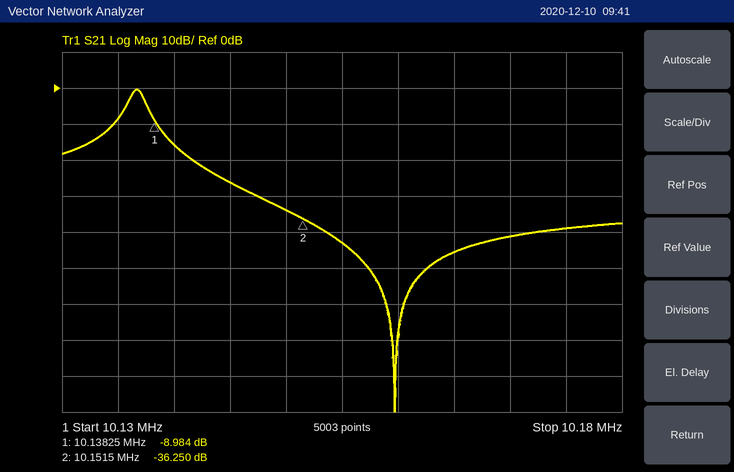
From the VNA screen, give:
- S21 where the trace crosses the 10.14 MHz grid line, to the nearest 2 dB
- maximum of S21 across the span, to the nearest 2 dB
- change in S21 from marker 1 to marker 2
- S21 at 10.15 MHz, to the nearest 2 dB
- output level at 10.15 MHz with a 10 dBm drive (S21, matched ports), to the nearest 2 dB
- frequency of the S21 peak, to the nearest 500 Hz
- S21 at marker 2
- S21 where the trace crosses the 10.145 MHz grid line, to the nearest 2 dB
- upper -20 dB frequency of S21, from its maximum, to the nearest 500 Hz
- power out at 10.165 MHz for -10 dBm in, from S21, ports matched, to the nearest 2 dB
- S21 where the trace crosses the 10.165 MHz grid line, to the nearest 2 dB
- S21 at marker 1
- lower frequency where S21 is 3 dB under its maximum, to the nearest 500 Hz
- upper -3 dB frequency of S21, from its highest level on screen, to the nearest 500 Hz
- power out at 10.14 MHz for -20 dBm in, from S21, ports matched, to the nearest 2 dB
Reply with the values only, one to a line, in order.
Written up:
-16 dB
0 dB
-27.266 dB
-34 dB
-24 dBm
10.1365 MHz
-36.250 dB
-26 dB
10.1420 MHz
-56 dBm
-46 dB
-8.984 dB
10.1360 MHz
10.1375 MHz
-36 dBm
